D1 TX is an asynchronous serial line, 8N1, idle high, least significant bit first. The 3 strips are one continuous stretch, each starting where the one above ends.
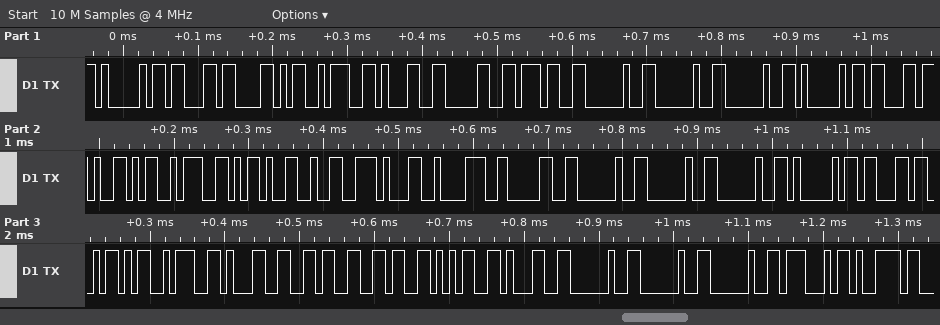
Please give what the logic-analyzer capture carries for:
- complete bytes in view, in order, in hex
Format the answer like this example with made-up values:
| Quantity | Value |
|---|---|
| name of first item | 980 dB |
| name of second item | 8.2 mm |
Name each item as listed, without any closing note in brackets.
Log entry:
| Quantity | Value |
|---|---|
| complete bytes in view, in order, in hex | 41 63 58 3A 31 30 37 20 20 20 41 63 59 3A 2D 32 31 38 30 20 20 20 41 63 5A 3A 31 36 36 35 31 20 20 20 47 79 |
